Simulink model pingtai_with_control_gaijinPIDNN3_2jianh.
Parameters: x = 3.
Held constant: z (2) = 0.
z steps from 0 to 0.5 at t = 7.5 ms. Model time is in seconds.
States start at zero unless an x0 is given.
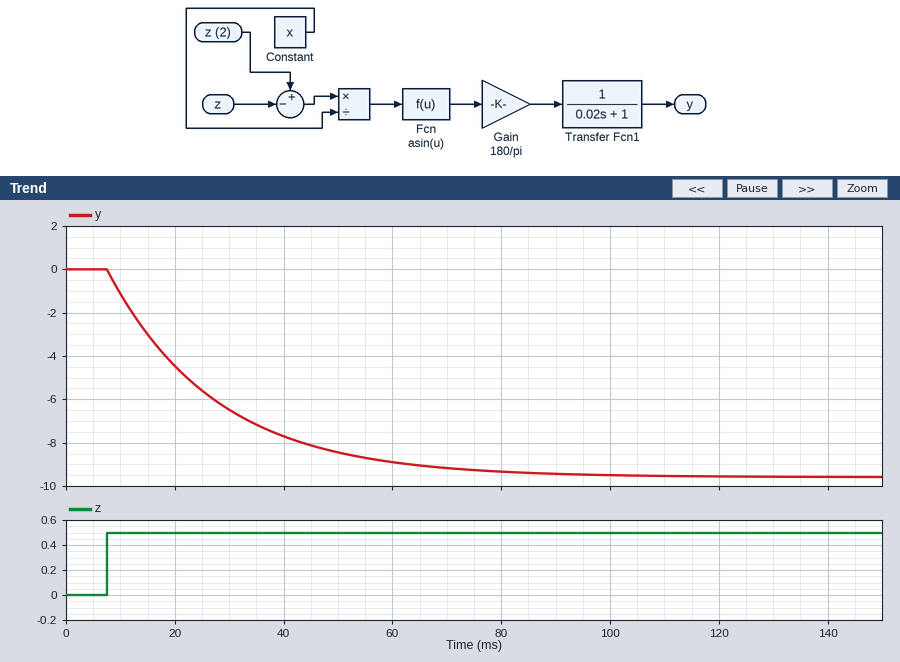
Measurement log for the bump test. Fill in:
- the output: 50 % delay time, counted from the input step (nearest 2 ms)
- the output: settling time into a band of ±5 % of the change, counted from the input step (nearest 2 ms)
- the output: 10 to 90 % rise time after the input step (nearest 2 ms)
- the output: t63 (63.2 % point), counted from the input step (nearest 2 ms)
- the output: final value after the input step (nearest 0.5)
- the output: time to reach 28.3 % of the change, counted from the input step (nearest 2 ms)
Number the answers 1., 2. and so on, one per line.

1. 14 ms
2. 60 ms
3. 44 ms
4. 20 ms
5. -9.5
6. 6 ms
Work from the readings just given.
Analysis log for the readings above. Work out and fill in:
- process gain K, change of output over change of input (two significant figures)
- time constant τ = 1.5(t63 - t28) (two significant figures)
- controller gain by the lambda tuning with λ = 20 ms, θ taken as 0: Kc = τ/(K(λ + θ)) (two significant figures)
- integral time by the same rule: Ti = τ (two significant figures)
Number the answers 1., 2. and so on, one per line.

1. -19
2. 21 ms
3. -0.055
4. 21 ms
